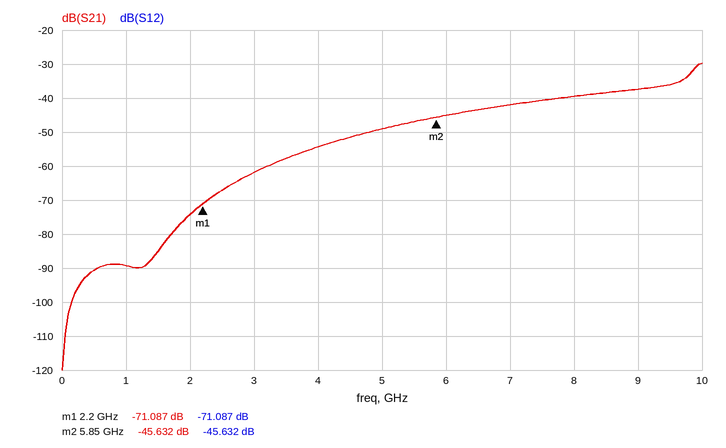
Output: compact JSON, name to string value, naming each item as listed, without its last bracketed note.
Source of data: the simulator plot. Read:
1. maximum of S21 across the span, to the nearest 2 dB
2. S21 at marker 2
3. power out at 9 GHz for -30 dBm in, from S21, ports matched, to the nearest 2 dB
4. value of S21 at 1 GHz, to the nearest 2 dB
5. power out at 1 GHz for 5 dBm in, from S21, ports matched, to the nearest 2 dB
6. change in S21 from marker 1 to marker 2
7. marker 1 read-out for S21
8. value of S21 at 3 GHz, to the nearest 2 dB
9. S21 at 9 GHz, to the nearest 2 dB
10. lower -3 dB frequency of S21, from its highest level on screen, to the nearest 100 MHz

{"maximum of S21 across the span, to the nearest 2 dB": "-30 dB", "S21 at marker 2": "-45.632 dB", "power out at 9 GHz for -30 dBm in, from S21, ports matched, to the nearest 2 dB": "-68 dBm", "value of S21 at 1 GHz, to the nearest 2 dB": "-90 dB", "power out at 1 GHz for 5 dBm in, from S21, ports matched, to the nearest 2 dB": "-84 dBm", "change in S21 from marker 1 to marker 2": "25.455 dB", "marker 1 read-out for S21": "-71.087 dB", "value of S21 at 3 GHz, to the nearest 2 dB": "-62 dB", "S21 at 9 GHz, to the nearest 2 dB": "-38 dB", "lower -3 dB frequency of S21, from its highest level on screen, to the nearest 100 MHz": "9.8 GHz"}
